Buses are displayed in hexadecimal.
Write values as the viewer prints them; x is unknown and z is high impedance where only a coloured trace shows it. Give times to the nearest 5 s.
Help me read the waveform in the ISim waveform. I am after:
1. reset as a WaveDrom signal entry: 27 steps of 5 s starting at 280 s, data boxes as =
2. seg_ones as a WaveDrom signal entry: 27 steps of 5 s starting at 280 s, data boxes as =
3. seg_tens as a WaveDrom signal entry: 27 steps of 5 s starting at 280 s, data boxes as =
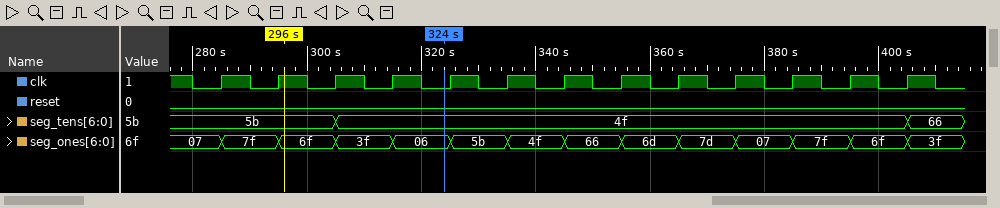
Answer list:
{name: 'reset', wave: '0..........................'}
{name: 'seg_ones', wave: '==.=.=.=.=.=.=.=.=.=.=.=.=.', data: '07 7f 6f 3f 06 5b 4f 66 6d 7d 07 7f 6f 3f'}
{name: 'seg_tens', wave: '=....=...................=.', data: '5b 4f 66'}
